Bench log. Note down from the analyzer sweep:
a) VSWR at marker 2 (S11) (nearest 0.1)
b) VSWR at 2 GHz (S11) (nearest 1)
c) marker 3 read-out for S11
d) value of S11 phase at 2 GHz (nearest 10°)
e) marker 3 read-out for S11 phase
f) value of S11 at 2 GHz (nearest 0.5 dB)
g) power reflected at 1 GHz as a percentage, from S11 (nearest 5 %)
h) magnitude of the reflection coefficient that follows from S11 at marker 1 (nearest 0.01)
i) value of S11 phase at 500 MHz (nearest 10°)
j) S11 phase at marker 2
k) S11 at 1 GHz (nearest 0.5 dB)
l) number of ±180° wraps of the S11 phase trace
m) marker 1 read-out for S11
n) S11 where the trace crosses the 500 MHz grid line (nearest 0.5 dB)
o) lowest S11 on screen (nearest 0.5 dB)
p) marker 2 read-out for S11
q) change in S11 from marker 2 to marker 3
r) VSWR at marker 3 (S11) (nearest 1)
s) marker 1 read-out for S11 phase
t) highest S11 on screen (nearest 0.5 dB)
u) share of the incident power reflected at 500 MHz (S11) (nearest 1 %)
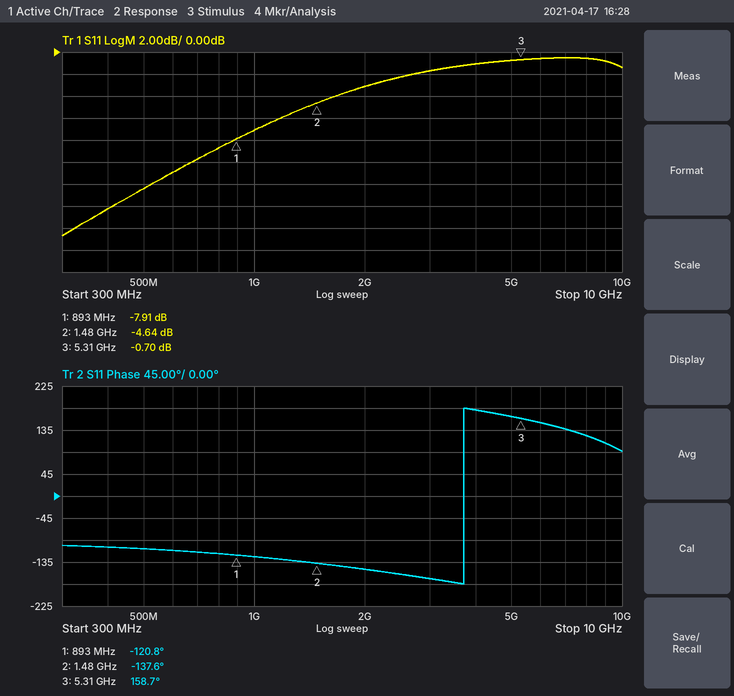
3.8
6
-0.70 dB
-150°
158.7°
-3.0 dB
20 %
0.40
-110°
-137.6°
-7.0 dB
1
-7.91 dB
-12.5 dB
-16.5 dB
-4.64 dB
3.94 dB
25
-120.8°
-0.5 dB
6 %
